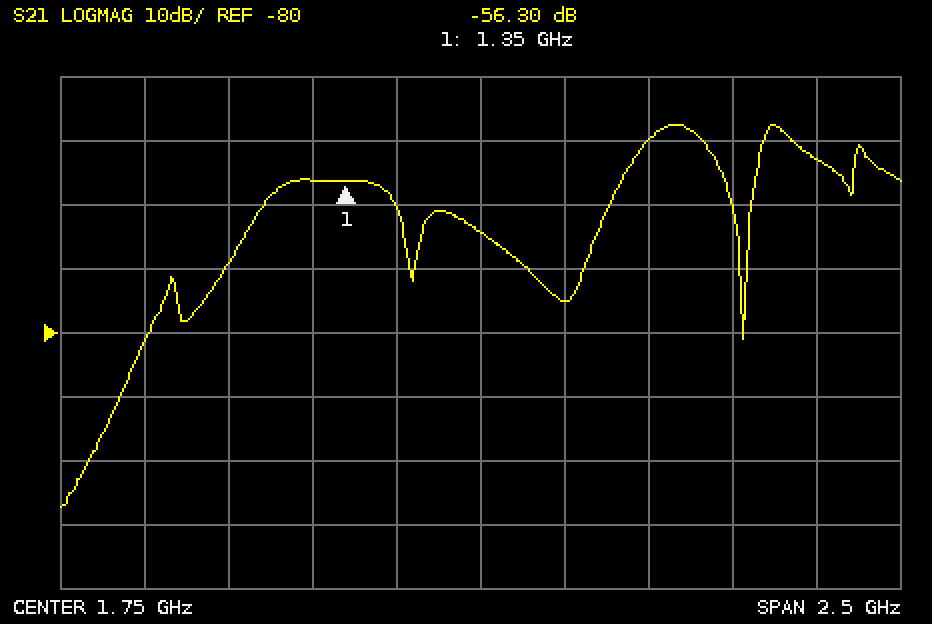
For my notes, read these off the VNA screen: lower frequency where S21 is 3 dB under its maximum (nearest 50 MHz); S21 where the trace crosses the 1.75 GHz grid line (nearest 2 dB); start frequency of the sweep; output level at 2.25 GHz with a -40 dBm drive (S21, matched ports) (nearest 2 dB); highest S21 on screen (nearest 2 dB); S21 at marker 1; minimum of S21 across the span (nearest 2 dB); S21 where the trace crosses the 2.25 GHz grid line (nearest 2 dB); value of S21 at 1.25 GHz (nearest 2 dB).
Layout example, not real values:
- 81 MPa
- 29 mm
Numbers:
- 2.25 GHz
- -64 dB
- 500 MHz
- -90 dBm
- -48 dB
- -56.30 dB
- -108 dB
- -50 dB
- -56 dB
